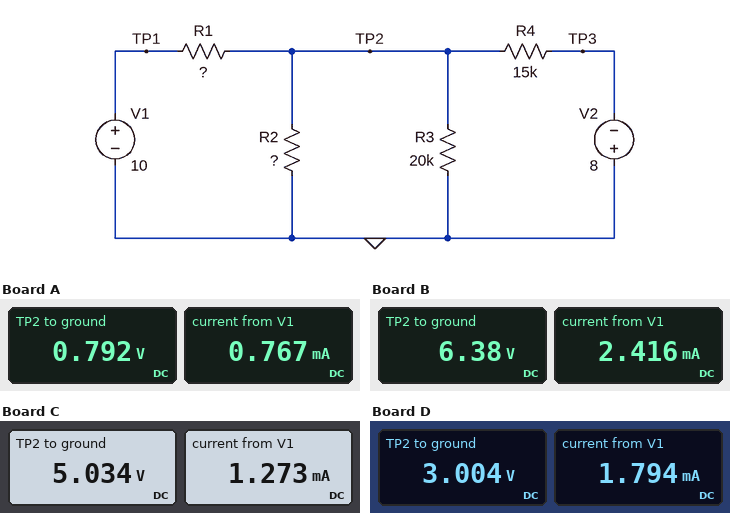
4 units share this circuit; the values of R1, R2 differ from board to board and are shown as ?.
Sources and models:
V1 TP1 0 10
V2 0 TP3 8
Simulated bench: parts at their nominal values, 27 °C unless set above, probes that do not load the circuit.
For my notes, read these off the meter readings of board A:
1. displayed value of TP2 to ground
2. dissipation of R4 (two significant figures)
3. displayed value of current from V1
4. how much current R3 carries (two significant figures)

0.792 V
5.2 mW
0.767 mA
40 µA
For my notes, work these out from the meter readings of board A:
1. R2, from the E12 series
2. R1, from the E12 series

5.6 kΩ
12 kΩ
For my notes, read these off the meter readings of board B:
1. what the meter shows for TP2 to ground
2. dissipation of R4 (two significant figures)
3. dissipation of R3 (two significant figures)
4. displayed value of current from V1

6.38 V
14 mW
2.0 mW
2.416 mA
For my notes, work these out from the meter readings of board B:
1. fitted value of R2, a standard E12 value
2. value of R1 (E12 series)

5.6 kΩ
1.5 kΩ
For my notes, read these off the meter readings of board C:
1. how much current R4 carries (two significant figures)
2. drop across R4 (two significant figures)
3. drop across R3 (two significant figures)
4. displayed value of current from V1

870 µA
13 V
5.0 V
1.273 mA
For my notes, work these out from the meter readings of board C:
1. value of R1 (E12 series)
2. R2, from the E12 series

3.9 kΩ
33 kΩ
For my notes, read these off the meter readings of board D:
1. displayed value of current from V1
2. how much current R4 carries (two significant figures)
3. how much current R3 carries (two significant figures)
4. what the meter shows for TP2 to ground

1.794 mA
730 µA
150 µA
3.004 V
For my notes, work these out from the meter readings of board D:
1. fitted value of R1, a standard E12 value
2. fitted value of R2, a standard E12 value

3.9 kΩ
3.3 kΩ
